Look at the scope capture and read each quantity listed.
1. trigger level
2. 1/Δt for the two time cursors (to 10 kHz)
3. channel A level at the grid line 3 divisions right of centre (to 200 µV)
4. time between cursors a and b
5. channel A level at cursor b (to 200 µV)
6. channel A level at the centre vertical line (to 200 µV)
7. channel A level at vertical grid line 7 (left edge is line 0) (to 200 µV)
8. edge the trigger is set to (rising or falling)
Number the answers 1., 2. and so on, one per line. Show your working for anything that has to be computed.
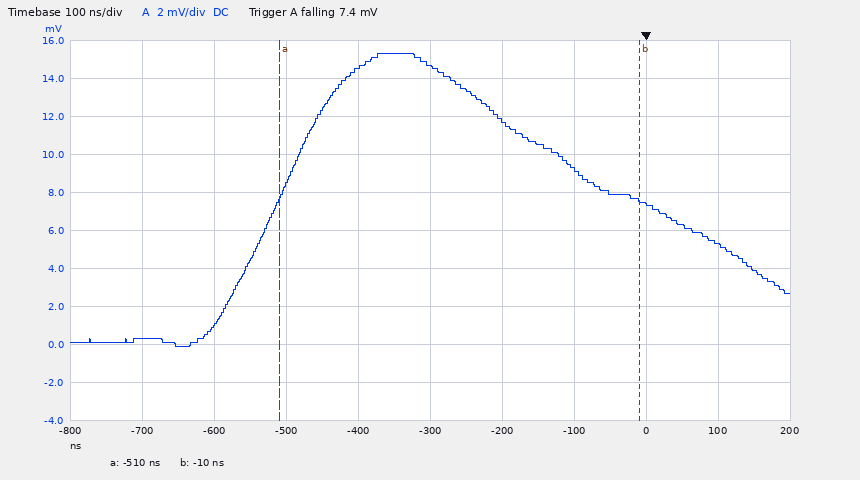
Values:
1. 7.4 mV
2. 1 / 500 ns ≈ 2.00 MHz
3. 7.4 mV
4. -10 ns − (-510 ns) = 500 ns
5. 7.6 mV
6. 14.6 mV
7. 9.2 mV
8. falling
